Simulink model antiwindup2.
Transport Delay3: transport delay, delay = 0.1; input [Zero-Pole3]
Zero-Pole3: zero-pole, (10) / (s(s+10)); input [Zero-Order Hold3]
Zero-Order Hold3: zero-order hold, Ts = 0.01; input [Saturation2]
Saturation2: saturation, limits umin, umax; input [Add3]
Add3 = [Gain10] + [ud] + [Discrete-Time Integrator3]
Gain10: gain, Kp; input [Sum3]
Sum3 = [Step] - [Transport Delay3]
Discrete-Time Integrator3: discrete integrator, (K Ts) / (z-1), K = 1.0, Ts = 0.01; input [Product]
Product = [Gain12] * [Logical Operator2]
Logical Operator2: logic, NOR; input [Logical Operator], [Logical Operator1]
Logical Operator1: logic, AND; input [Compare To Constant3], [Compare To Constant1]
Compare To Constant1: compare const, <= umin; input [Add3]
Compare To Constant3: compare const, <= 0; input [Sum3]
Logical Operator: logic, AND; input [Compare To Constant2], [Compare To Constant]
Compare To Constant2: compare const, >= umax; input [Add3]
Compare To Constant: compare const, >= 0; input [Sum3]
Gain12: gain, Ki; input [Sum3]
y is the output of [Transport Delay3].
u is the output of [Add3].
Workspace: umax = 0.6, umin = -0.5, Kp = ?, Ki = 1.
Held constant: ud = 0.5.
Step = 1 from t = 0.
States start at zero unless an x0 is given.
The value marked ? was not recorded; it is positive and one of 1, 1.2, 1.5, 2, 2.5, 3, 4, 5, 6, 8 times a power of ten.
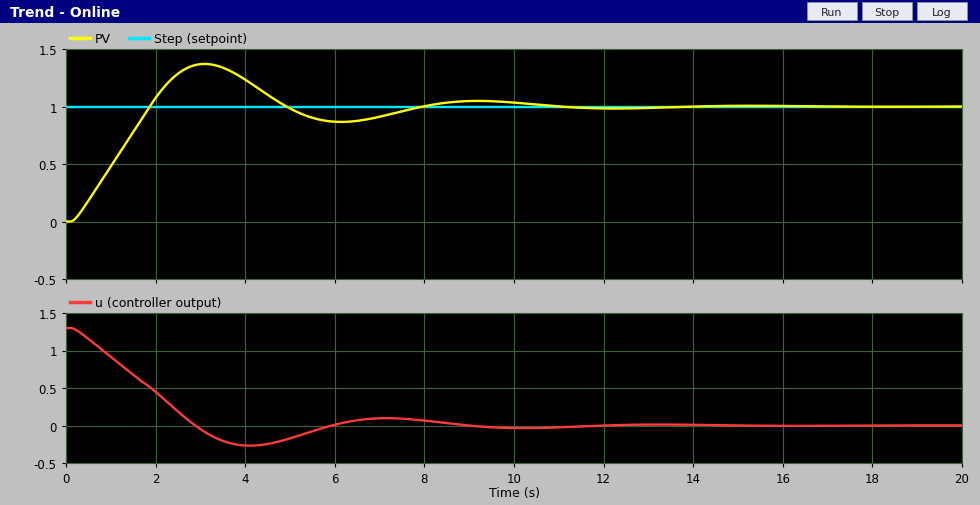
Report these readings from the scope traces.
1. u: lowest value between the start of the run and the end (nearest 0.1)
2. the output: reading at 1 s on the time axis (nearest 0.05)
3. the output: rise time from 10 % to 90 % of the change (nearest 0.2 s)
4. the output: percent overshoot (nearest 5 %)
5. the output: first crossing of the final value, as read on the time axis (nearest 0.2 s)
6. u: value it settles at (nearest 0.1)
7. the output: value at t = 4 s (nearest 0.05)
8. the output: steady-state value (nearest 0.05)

-0.3
0.50
1.4 s
35 %
1.8 s
0.0
1.25
1.00
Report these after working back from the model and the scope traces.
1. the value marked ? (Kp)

0.8
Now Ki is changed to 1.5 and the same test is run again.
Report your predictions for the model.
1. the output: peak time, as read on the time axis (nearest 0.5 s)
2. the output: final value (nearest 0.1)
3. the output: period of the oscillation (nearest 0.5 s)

3.0 s
1.0
5.0 s
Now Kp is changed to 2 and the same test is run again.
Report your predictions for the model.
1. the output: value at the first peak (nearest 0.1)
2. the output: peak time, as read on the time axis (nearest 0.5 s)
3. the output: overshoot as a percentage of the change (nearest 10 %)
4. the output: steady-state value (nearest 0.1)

1.2
2.5 s
20 %
1.0
